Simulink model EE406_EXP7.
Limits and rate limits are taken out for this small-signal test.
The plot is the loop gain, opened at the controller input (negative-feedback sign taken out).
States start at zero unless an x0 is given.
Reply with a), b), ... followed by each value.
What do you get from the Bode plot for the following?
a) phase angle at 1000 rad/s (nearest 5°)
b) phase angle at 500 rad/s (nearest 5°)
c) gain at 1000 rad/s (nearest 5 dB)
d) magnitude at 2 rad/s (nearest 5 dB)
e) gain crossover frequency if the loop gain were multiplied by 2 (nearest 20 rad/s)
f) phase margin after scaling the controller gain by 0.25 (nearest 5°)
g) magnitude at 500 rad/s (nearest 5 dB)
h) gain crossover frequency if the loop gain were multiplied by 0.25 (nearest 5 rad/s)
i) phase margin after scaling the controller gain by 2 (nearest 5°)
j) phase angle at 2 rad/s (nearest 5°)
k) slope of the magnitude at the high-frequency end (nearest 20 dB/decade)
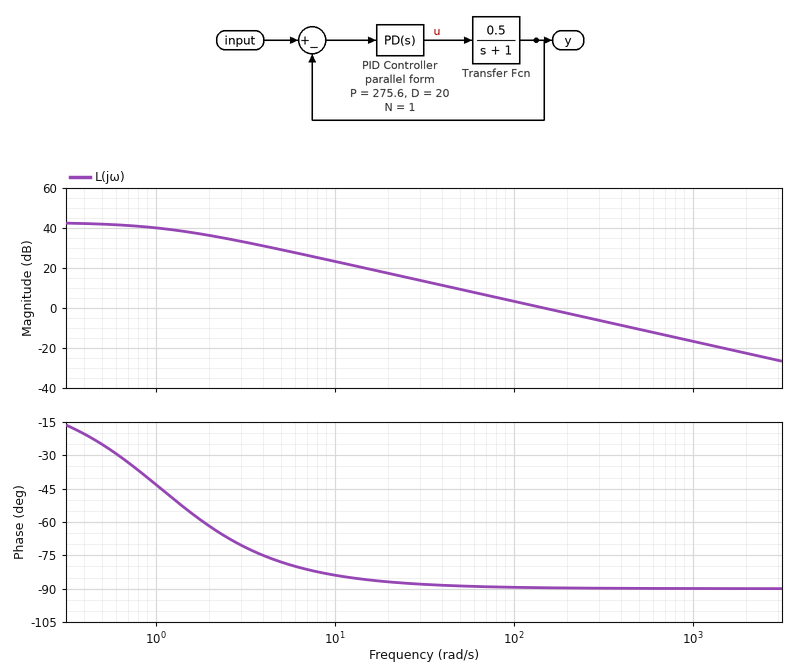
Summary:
a) -90°
b) -90°
c) -15 dB
d) 35 dB
e) 300 rad/s
f) 90°
g) -10 dB
h) 35 rad/s
i) 90°
j) -60°
k) -20 dB/decade
